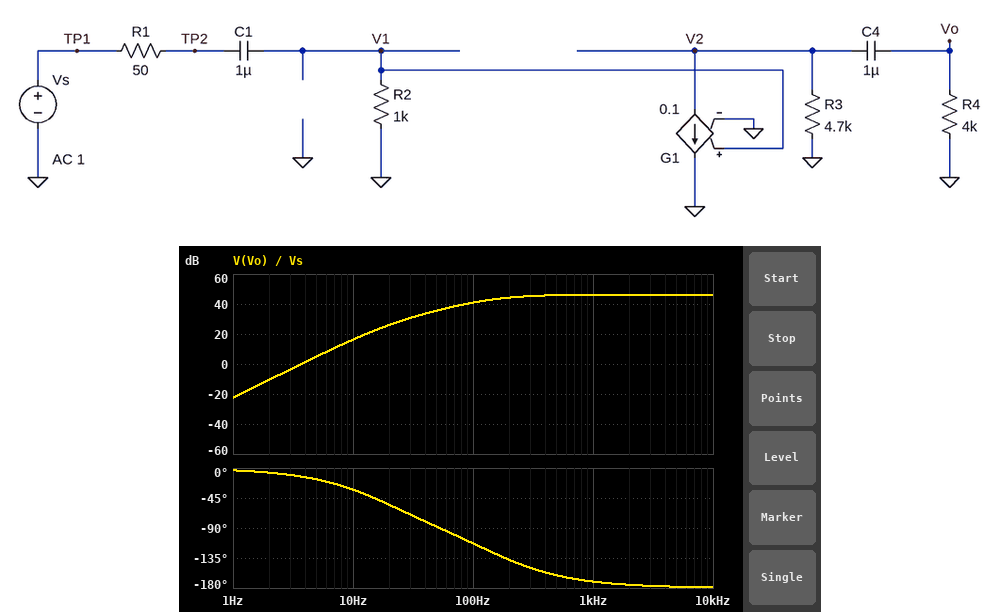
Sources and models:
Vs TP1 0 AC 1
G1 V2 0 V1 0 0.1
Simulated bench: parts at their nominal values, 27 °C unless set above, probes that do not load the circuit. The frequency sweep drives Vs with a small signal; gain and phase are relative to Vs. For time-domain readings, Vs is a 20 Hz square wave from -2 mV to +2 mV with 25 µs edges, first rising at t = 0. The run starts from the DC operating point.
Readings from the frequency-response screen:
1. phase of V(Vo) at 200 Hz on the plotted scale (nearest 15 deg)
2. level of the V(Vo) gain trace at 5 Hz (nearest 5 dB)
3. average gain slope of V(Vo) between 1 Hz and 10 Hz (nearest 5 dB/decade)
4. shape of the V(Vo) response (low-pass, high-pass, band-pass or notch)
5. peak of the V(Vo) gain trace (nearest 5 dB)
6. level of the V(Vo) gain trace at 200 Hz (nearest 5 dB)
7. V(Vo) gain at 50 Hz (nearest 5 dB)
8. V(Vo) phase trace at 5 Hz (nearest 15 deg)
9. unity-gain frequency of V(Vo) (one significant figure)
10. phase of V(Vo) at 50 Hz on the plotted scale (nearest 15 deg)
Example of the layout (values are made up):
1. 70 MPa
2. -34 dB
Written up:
1. -135 deg
2. 5 dB
3. 40 dB/decade
4. high-pass
5. 45 dB
6. 45 dB
7. 35 dB
8. -15 deg
9. 4 Hz
10. -90 deg
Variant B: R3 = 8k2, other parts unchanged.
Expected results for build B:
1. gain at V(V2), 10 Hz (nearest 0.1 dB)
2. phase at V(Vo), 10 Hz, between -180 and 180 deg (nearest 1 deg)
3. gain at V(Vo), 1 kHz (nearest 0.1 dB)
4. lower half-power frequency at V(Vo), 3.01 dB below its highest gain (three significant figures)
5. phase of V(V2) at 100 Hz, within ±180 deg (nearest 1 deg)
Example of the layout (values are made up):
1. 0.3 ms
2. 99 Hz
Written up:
1. 32.5 dB
2. -41 deg
3. 48.1 dB
4. 153 Hz
5. -138 deg
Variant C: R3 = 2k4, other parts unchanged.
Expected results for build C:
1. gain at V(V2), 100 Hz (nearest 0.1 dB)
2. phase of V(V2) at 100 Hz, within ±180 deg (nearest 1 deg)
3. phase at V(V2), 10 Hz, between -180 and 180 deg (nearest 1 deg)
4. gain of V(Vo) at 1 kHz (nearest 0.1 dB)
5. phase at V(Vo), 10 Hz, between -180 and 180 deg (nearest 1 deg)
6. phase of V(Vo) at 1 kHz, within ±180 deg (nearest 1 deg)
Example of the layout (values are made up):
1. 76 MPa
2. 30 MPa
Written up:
1. 38.3 dB
2. -131 deg
3. -102 deg
4. 43.0 dB
5. -26 deg
6. -170 deg
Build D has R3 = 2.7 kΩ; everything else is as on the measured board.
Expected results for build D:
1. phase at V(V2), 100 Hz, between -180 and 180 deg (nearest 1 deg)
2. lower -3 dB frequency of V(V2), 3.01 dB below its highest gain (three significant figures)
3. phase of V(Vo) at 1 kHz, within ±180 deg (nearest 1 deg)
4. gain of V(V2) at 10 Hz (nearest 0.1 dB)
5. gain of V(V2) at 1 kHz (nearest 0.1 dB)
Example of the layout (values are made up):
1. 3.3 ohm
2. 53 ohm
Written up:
1. -132 deg
2. 145 Hz
3. -170 deg
4. 24.1 dB
5. 43.6 dB
